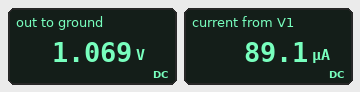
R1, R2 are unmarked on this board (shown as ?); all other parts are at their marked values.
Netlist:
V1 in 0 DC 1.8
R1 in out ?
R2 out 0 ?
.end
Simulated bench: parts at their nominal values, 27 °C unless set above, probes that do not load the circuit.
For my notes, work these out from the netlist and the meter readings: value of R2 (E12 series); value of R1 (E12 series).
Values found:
12 kΩ
8.2 kΩ
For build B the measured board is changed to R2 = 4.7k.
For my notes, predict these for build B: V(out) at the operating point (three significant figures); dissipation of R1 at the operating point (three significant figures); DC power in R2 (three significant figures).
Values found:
656 mV
160 µW
91.5 µW
